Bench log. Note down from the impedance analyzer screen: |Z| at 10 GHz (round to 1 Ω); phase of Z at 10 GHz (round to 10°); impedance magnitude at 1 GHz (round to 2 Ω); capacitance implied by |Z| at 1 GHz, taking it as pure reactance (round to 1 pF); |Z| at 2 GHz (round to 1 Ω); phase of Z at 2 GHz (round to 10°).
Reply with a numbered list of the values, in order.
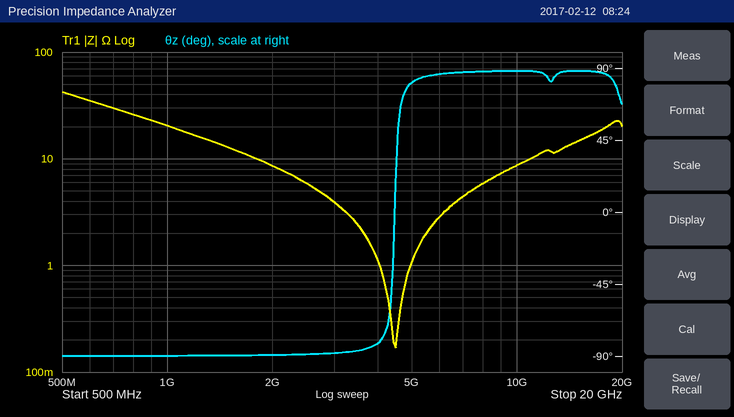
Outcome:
1. 9 Ω
2. 90°
3. 20 Ω
4. 8 pF
5. 9 Ω
6. -90°
